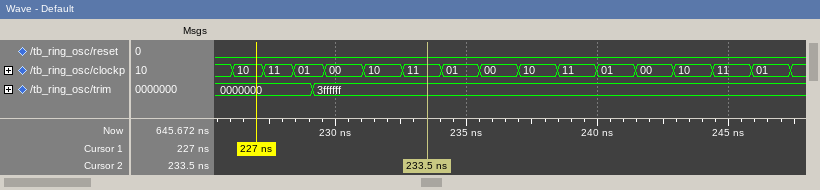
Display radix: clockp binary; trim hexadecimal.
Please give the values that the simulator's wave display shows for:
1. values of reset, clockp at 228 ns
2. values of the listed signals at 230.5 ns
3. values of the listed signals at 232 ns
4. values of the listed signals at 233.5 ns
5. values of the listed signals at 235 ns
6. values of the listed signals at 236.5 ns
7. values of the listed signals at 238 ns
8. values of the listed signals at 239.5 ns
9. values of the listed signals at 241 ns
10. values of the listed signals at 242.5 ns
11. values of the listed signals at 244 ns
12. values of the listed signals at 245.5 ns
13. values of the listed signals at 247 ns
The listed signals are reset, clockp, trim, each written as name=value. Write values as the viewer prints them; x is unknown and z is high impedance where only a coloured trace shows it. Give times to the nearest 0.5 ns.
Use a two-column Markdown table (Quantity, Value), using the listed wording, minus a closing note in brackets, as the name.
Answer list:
| Quantity | Value |
|---|---|
| values of reset, clockp at 228 ns | reset=0, clockp=11 |
| values of the listed signals at 230.5 ns | reset=0, clockp=00, trim=3ffffff |
| values of the listed signals at 232 ns | reset=0, clockp=10, trim=3ffffff |
| values of the listed signals at 233.5 ns | reset=0, clockp=11, trim=3ffffff |
| values of the listed signals at 235 ns | reset=0, clockp=01, trim=3ffffff |
| values of the listed signals at 236.5 ns | reset=0, clockp=00, trim=3ffffff |
| values of the listed signals at 238 ns | reset=0, clockp=10, trim=3ffffff |
| values of the listed signals at 239.5 ns | reset=0, clockp=11, trim=3ffffff |
| values of the listed signals at 241 ns | reset=0, clockp=01, trim=3ffffff |
| values of the listed signals at 242.5 ns | reset=0, clockp=00, trim=3ffffff |
| values of the listed signals at 244 ns | reset=0, clockp=10, trim=3ffffff |
| values of the listed signals at 245.5 ns | reset=0, clockp=11, trim=3ffffff |
| values of the listed signals at 247 ns | reset=0, clockp=01, trim=3ffffff |
